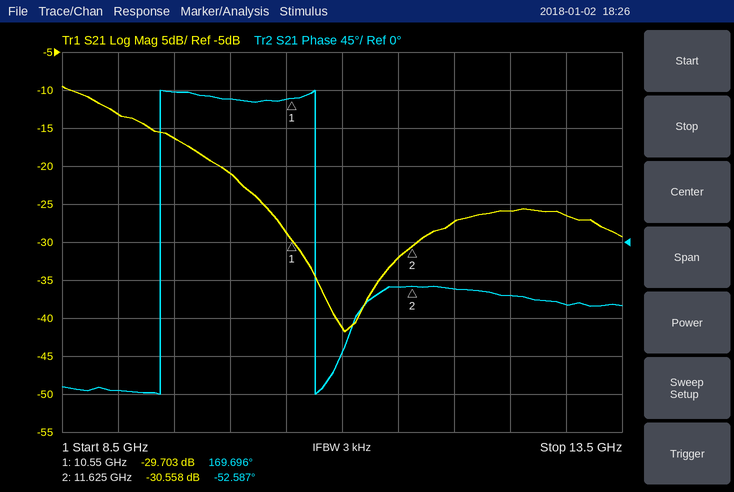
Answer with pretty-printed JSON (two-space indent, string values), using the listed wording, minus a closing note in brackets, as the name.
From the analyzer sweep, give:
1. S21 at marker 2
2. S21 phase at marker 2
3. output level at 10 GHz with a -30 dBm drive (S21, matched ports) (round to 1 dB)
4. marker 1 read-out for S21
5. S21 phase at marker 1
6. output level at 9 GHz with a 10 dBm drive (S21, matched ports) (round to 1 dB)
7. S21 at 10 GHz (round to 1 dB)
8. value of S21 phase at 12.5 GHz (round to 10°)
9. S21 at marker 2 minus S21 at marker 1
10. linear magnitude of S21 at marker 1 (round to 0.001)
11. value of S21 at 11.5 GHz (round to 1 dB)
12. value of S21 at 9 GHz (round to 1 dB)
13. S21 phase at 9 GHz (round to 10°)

{
  "S21 at marker 2": "-30.558 dB",
  "S21 phase at marker 2": "-52.587°",
  "output level at 10 GHz with a -30 dBm drive (S21, matched ports)": "-51 dBm",
  "marker 1 read-out for S21": "-29.703 dB",
  "S21 phase at marker 1": "169.696°",
  "output level at 9 GHz with a 10 dBm drive (S21, matched ports)": "-3 dBm",
  "S21 at 10 GHz": "-21 dB",
  "value of S21 phase at 12.5 GHz": "-60°",
  "S21 at marker 2 minus S21 at marker 1": "-0.855 dB",
  "linear magnitude of S21 at marker 1": "0.033",
  "value of S21 at 11.5 GHz": "-32 dB",
  "value of S21 at 9 GHz": "-13 dB",
  "S21 phase at 9 GHz": "-180°"
}
